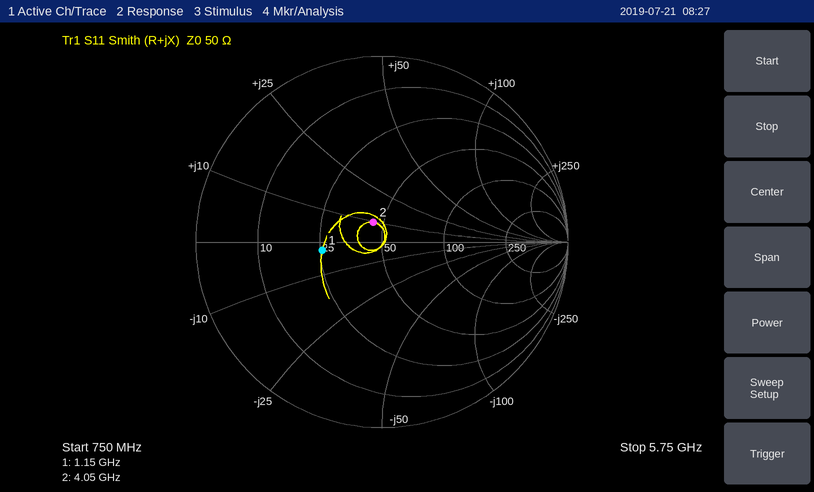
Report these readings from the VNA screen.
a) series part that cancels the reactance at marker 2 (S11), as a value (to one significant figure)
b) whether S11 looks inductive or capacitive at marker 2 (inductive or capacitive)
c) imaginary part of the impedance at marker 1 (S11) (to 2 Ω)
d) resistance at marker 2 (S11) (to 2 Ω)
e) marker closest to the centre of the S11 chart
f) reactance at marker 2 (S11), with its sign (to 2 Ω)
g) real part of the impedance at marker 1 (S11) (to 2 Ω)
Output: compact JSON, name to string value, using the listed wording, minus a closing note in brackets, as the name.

{"series part that cancels the reactance at marker 2 (S11), as a value": "4 pF", "whether S11 looks inductive or capacitive at marker 2": "inductive", "imaginary part of the impedance at marker 1 (S11)": "-2 Ω", "resistance at marker 2 (S11)": "44 Ω", "marker closest to the centre of the S11 chart": "marker 2", "reactance at marker 2 (S11), with its sign": "+10 Ω", "real part of the impedance at marker 1 (S11)": "26 Ω"}
